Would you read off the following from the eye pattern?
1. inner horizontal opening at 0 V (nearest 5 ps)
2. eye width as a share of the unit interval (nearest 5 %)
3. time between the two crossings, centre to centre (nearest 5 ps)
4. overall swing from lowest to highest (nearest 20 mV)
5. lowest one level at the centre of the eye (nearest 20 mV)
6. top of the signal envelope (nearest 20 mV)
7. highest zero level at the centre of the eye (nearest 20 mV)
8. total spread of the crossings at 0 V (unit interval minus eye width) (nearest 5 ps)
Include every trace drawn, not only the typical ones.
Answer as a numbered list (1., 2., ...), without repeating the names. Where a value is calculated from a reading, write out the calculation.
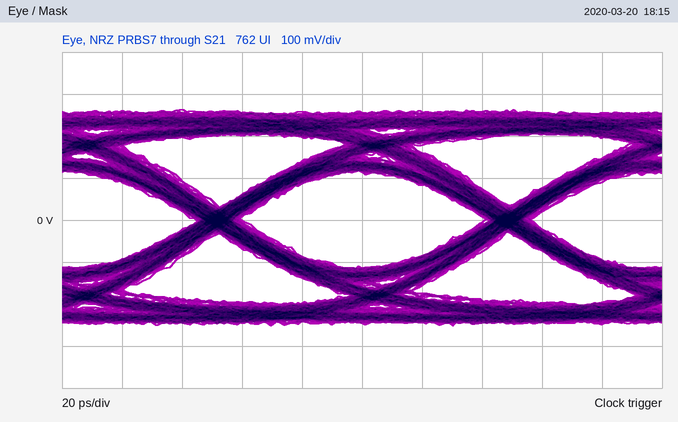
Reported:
1. 80 ps
2. 80 ps / 95 ps ≈ 84.2 %, so 85 % to the nearest 5 %
3. 95 ps
4. 520 mV
5. 120 mV
6. 260 mV
7. -120 mV
8. 15 ps
